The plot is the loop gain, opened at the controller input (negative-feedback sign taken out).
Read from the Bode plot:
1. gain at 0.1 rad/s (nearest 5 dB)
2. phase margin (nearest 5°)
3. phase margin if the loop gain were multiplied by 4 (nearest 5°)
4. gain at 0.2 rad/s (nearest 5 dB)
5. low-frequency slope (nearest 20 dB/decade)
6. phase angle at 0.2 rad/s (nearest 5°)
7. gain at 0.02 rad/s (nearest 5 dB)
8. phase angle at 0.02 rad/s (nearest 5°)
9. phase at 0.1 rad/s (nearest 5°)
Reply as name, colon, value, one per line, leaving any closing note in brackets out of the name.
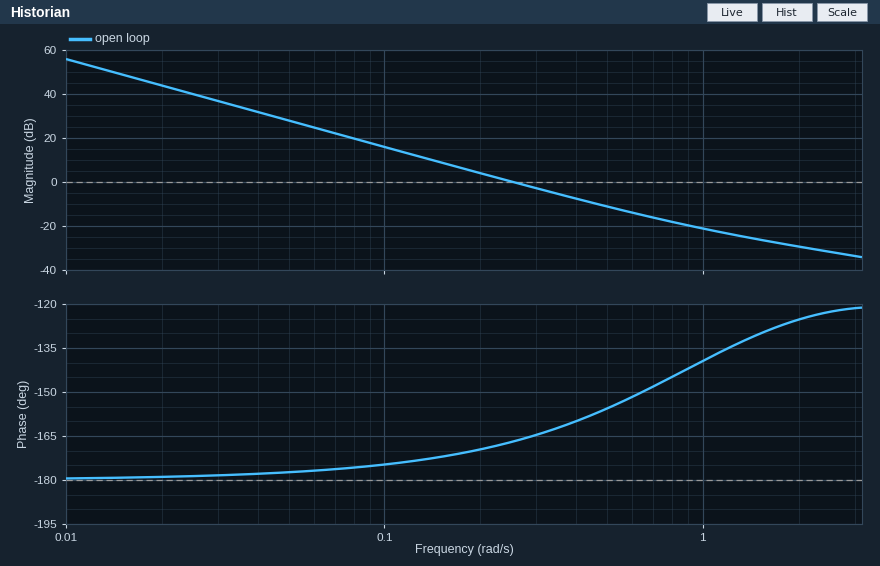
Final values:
gain at 0.1 rad/s: 15 dB
phase margin: 15°
phase margin if the loop gain were multiplied by 4: 25°
gain at 0.2 rad/s: 5 dB
low-frequency slope: -40 dB/decade
phase angle at 0.2 rad/s: -170°
gain at 0.02 rad/s: 45 dB
phase angle at 0.02 rad/s: -180°
phase at 0.1 rad/s: -175°
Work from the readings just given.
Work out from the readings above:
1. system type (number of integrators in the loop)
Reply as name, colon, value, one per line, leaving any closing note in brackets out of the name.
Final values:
system type: 2
